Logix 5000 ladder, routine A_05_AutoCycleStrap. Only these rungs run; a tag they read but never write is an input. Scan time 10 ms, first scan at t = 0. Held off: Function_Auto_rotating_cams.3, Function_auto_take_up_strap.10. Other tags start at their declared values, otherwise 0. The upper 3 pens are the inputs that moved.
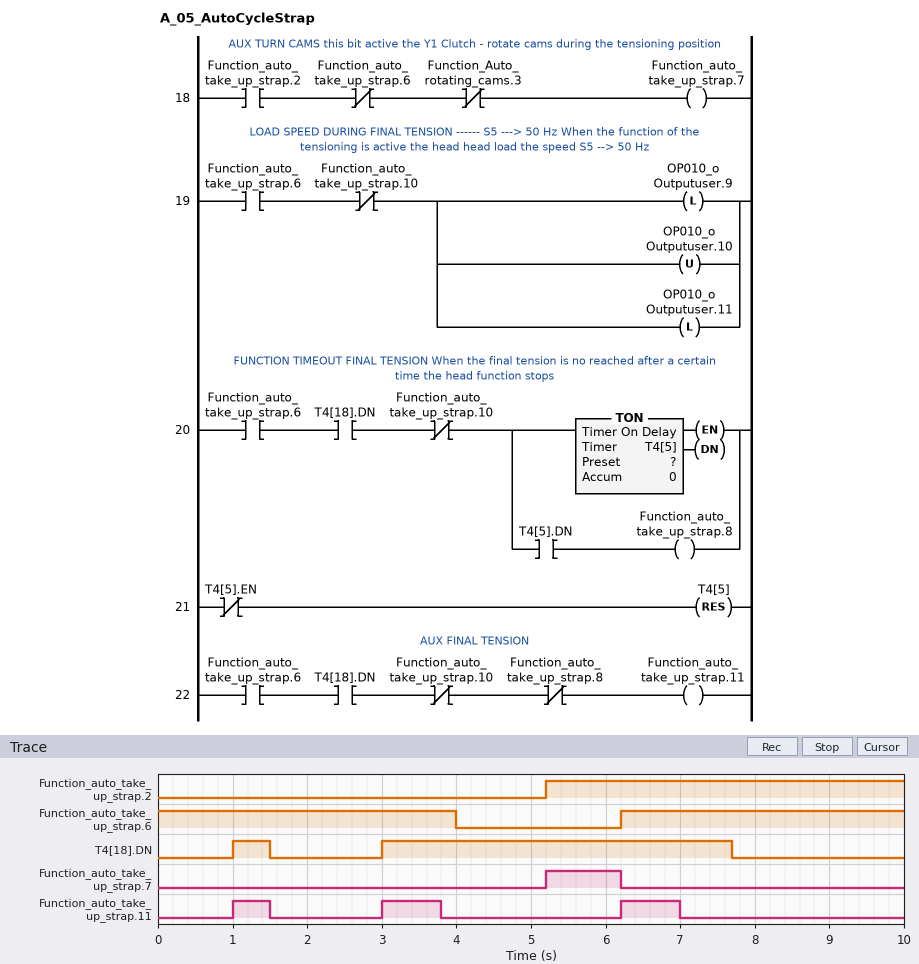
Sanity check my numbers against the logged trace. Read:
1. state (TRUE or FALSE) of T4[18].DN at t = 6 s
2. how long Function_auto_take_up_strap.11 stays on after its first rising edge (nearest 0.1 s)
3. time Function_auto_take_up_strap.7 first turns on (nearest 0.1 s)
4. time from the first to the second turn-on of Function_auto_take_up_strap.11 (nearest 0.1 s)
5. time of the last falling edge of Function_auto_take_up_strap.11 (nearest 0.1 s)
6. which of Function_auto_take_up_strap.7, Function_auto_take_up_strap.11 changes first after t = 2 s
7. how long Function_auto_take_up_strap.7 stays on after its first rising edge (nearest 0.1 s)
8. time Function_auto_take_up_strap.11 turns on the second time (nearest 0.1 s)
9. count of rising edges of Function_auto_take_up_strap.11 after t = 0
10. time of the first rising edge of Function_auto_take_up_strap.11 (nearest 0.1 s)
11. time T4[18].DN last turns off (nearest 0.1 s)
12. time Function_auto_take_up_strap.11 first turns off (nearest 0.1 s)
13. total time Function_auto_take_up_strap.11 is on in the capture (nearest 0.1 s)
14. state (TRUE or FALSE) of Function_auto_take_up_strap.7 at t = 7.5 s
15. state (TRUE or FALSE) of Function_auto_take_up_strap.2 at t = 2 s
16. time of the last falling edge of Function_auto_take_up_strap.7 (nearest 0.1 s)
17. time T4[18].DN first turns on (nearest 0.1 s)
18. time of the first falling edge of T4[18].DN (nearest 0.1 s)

TRUE
0.5 s
5.2 s
2.0 s
7.0 s
Function_auto_take_up_strap.11
1.0 s
3.0 s
3
1.0 s
7.7 s
1.5 s
2.1 s
FALSE
FALSE
6.2 s
1.0 s
1.5 s
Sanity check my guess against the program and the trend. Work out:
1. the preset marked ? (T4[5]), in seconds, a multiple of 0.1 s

0.8 s
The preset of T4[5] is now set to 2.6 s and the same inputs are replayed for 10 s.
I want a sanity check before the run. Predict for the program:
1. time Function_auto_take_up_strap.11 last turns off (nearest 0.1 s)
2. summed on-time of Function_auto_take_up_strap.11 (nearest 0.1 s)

7.7 s
3.0 s
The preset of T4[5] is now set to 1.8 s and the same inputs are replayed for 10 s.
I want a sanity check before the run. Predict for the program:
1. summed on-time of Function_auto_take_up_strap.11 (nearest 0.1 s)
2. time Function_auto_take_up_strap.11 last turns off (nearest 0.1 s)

3.0 s
7.7 s
